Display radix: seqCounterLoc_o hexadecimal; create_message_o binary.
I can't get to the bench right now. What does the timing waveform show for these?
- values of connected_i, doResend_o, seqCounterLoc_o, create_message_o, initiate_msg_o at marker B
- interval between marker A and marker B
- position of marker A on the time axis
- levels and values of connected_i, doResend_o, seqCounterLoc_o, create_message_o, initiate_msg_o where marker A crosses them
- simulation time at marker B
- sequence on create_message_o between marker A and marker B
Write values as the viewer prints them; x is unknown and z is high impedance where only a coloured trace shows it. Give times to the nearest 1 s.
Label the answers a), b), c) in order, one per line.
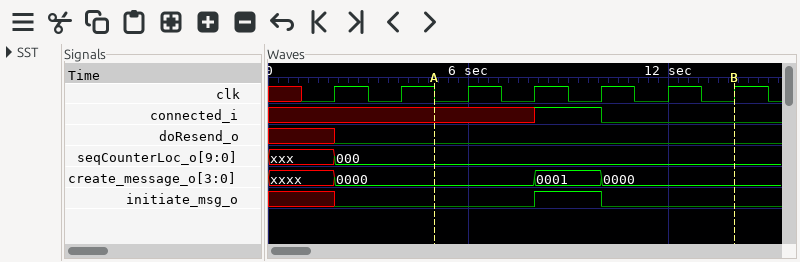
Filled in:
a) connected_i=0, doResend_o=0, seqCounterLoc_o=000, create_message_o=0000, initiate_msg_o=0
b) 9 s
c) 5 s
d) connected_i=x, doResend_o=0, seqCounterLoc_o=000, create_message_o=0000, initiate_msg_o=0
e) 14 s
f) 0000, 0001, 0000
